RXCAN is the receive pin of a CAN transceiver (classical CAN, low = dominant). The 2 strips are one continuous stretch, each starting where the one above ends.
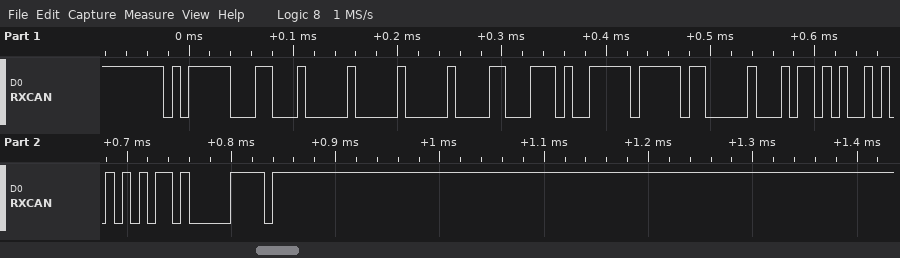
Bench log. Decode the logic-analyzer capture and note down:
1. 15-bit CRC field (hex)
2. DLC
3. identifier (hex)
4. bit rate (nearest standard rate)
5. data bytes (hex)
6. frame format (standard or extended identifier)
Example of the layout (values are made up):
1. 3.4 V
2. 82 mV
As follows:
1. 0x5683
2. 8
3. 0x5F3
4. 125 kbit/s
5. 00 00 C7 4F FF 00 B5 2A
6. standard
